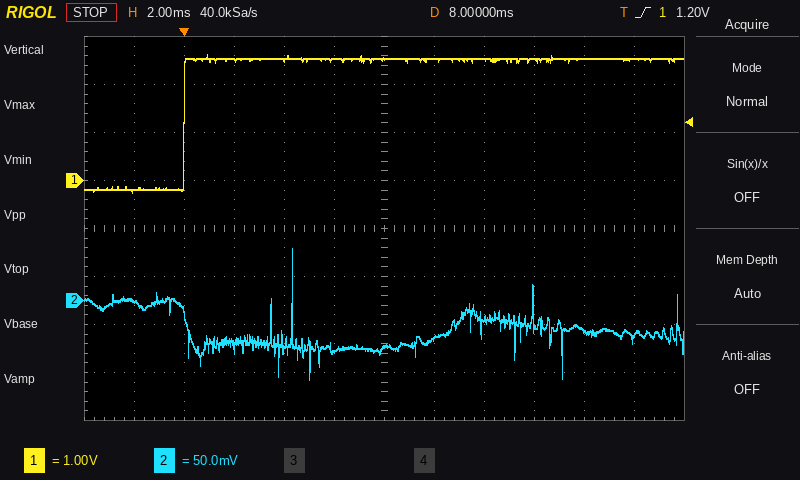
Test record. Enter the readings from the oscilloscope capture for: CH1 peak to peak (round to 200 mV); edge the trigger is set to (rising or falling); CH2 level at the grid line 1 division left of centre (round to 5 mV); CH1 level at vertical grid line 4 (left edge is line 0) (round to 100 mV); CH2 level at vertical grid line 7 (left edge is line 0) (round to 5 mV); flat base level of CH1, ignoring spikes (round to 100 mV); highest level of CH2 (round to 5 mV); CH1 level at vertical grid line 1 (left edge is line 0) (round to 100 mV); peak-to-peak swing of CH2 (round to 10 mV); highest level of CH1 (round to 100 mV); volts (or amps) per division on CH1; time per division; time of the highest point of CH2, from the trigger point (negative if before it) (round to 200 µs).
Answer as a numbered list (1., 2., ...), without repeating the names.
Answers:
1. 2.8 V
2. rising
3. -55 mV
4. 2.5 V
5. -40 mV
6. -200 mV
7. 55 mV
8. -200 mV
9. 140 mV
10. 2.6 V
11. 1 V
12. 2 ms
13. +4.4 ms
